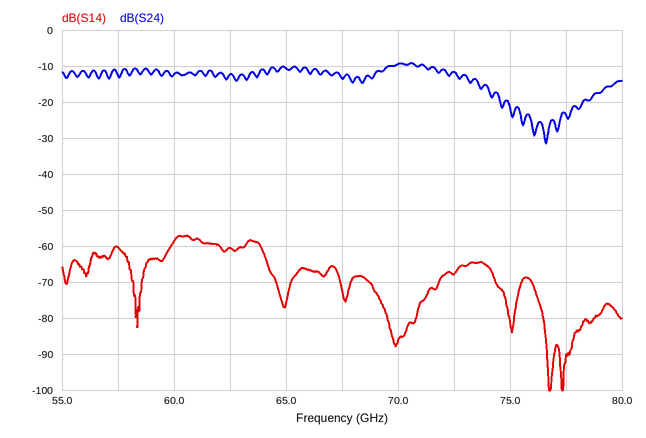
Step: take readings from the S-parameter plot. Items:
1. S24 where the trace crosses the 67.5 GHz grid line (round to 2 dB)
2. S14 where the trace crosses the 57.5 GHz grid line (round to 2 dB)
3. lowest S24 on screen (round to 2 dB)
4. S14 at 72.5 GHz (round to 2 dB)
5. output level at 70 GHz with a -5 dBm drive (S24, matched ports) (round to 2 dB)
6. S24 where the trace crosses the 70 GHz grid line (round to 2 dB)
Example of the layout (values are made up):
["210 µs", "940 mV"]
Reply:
["-14 dB", "-60 dB", "-32 dB", "-68 dB", "-14 dBm", "-10 dB"]
